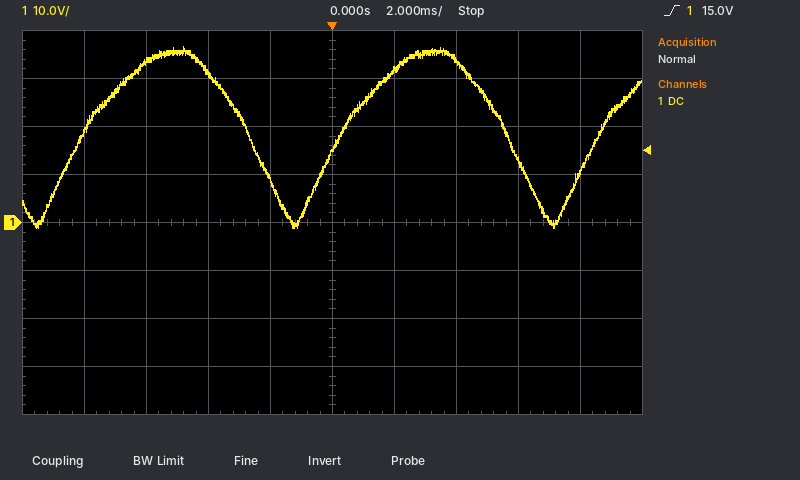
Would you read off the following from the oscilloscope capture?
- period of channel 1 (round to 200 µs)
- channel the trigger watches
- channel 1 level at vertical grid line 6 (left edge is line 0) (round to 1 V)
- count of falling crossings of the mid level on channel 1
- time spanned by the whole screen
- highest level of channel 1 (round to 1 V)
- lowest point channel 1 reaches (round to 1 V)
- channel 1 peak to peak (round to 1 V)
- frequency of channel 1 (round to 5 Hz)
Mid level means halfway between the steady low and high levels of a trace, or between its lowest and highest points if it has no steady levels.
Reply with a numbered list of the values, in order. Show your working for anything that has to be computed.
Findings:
1. 8.4 ms
2. channel 1
3. 32 V
4. 2
5. 20 ms
6. 37 V
7. -1 V
8. 37 V − (-1 V) = 38 V
9. 1 / 8.4 ms ≈ 119 Hz, so 120 Hz to the nearest 5 Hz
